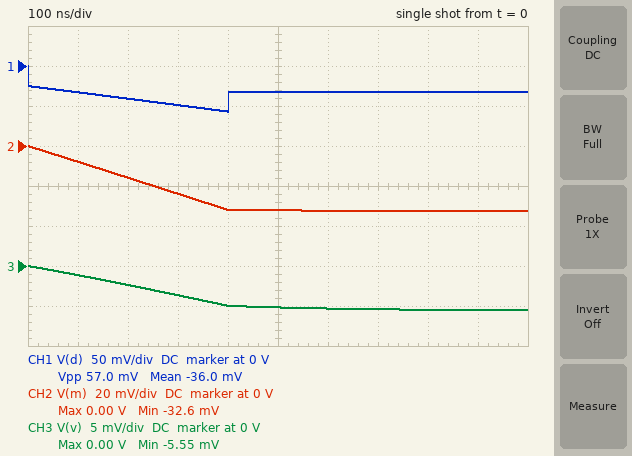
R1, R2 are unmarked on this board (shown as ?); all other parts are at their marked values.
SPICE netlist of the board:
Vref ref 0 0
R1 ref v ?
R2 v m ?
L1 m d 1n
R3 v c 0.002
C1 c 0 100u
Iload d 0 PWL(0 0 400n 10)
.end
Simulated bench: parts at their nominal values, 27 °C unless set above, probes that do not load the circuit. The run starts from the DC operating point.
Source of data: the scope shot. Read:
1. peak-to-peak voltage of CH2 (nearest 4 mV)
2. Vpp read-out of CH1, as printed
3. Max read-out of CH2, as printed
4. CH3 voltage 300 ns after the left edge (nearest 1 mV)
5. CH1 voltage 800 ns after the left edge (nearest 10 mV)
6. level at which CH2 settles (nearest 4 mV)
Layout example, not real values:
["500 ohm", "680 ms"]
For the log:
["32 mV", "57.0 mV", "0.00 V", "-4 mV", "-30 mV", "-32 mV"]
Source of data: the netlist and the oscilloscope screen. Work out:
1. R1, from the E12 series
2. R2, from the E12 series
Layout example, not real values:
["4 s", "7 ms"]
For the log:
["560 µΩ", "2.7 mΩ"]
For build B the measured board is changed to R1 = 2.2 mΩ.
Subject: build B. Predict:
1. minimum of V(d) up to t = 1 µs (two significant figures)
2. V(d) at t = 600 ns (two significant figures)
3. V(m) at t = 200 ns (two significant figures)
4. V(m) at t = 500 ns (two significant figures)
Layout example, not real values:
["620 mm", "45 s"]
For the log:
["-67 mV", "-44 mV", "-20 mV", "-43 mV"]
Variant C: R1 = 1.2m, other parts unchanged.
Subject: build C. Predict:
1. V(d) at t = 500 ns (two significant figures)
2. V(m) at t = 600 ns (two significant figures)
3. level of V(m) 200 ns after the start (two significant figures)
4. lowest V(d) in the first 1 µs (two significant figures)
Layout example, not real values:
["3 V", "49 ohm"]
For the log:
["-37 mV", "-38 mV", "-18 mV", "-61 mV"]
